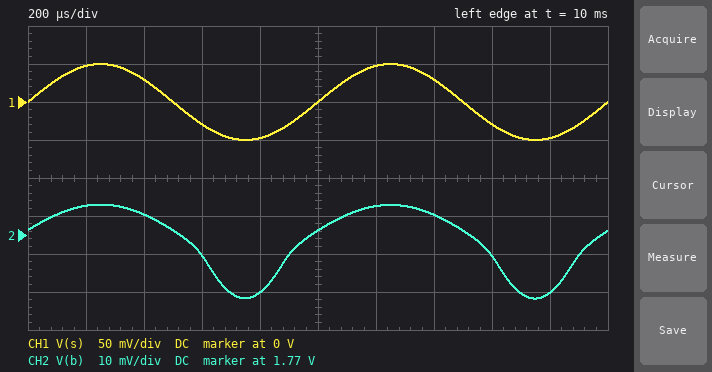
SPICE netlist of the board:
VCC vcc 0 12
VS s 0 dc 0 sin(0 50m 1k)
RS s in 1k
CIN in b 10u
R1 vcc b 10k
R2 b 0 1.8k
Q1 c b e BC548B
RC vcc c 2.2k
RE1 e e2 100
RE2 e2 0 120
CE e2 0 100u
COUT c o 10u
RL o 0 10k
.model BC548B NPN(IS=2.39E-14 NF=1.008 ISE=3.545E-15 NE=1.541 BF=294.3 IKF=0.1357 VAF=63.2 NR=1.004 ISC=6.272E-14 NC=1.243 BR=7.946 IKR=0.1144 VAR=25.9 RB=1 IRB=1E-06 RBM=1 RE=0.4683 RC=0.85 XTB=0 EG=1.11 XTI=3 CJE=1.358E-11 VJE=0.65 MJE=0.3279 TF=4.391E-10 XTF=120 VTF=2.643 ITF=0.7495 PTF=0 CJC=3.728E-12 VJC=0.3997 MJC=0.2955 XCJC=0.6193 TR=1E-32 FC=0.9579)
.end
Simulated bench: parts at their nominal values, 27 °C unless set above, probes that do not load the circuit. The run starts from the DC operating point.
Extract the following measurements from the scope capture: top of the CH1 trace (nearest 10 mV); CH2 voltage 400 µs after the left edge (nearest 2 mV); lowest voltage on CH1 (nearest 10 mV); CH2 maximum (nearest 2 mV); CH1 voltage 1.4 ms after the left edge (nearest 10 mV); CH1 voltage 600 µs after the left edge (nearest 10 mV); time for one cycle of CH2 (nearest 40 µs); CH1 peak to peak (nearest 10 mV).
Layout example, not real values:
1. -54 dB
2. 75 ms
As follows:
1. 50 mV
2. 1.776 V
3. -50 mV
4. 1.778 V
5. 30 mV
6. -30 mV
7. 1.00 ms
8. 100 mV
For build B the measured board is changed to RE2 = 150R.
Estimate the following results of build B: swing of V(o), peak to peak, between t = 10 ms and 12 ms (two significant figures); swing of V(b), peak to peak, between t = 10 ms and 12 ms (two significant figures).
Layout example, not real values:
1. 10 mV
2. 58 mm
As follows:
1. 990 mV
2. 59 mV
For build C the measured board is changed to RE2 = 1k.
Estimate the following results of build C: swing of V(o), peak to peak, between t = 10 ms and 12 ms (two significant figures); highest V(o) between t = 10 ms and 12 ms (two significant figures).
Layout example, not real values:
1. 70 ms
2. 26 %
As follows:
1. 850 mV
2. 420 mV
